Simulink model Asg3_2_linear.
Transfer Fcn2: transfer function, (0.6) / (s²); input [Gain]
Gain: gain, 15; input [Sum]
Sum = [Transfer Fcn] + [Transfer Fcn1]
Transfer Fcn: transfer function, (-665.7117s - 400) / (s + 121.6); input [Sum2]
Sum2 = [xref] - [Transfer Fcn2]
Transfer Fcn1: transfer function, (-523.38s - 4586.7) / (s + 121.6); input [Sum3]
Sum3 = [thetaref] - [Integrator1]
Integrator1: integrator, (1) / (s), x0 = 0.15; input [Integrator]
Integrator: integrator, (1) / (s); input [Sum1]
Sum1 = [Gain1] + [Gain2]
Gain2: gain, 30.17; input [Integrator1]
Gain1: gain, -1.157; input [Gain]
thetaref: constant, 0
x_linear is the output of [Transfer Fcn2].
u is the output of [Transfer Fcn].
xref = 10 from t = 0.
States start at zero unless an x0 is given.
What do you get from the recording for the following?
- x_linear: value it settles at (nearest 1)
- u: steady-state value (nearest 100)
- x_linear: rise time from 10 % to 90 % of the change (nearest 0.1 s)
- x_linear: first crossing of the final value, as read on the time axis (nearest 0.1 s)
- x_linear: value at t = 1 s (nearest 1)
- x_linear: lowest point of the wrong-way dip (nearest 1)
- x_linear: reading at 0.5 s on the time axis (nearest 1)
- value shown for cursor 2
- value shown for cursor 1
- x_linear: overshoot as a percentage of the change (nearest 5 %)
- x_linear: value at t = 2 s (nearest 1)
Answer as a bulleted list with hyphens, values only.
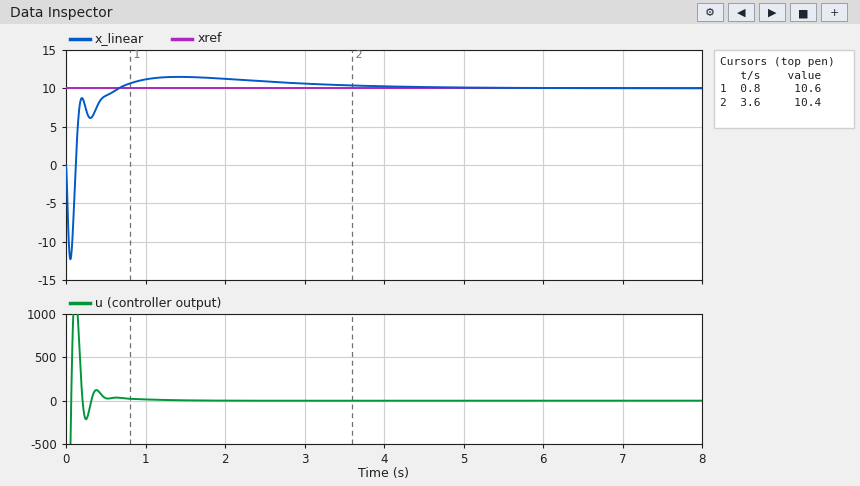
- 10
- 0
- 0.4 s
- 0.7 s
- 11
- -12
- 9
- 10.4
- 10.6
- 15 %
- 11
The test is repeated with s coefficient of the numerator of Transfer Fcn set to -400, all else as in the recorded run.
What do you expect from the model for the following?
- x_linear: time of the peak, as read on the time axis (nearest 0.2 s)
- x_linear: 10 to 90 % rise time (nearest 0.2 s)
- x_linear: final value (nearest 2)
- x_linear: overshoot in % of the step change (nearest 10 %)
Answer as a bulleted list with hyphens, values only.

- 1.8 s
- 0.6 s
- 10
- 30 %
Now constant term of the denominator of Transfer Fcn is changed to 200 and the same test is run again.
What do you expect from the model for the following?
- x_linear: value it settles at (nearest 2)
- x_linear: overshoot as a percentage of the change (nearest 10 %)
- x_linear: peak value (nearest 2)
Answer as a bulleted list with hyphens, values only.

- 10
- 20 %
- 12
